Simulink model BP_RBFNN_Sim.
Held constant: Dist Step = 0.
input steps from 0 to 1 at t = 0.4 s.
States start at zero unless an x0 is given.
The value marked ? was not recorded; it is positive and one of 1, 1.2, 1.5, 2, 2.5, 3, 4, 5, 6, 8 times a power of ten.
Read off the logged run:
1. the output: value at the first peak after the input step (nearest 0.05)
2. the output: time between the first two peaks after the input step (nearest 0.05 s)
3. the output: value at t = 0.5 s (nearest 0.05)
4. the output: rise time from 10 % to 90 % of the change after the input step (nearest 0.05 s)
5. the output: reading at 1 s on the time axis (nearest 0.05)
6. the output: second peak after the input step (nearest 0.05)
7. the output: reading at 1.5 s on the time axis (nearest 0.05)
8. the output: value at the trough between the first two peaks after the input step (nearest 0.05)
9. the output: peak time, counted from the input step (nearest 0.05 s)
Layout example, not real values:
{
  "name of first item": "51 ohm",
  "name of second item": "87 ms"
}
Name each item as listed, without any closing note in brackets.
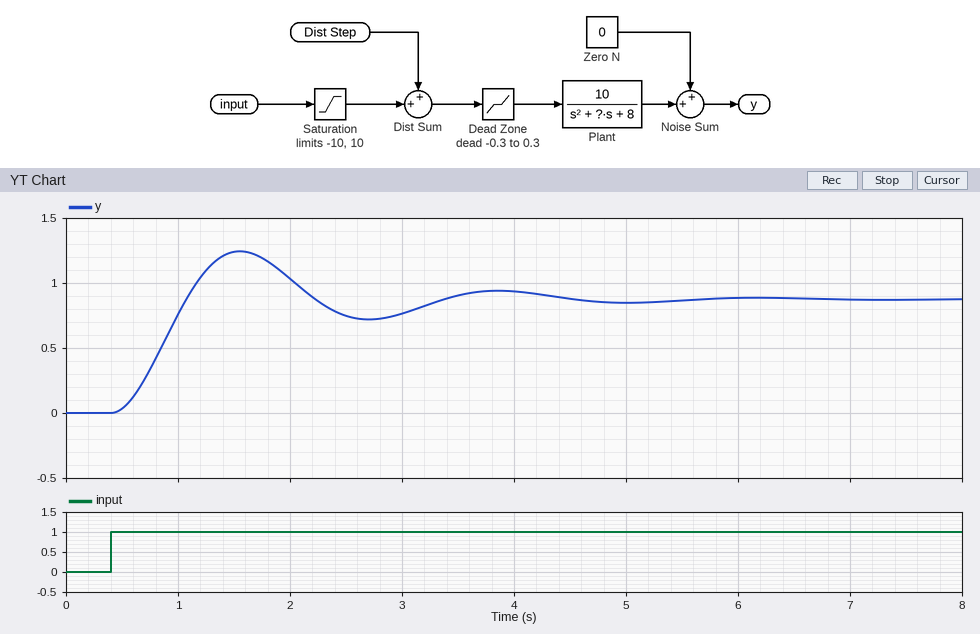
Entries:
{
  "the output: value at the first peak after the input step": "1.25",
  "the output: time between the first two peaks after the input step": "2.30 s",
  "the output: value at t = 0.5 s": "0.05",
  "the output: rise time from 10 % to 90 % of the change after the input step": "0.45 s",
  "the output: reading at 1 s on the time axis": "0.75",
  "the output: second peak after the input step": "0.95",
  "the output: reading at 1.5 s on the time axis": "1.25",
  "the output: value at the trough between the first two peaks after the input step": "0.70",
  "the output: peak time, counted from the input step": "1.15 s"
}
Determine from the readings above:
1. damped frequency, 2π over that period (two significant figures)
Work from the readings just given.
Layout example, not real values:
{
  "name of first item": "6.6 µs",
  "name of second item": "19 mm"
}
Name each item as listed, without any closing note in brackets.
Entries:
{
  "damped frequency, 2π over that period": "2.7 rad/s"
}
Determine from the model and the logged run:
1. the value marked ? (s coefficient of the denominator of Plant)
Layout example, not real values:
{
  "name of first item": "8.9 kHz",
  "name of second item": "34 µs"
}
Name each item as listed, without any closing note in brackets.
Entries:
{
  "the value marked ?": "1.5"
}
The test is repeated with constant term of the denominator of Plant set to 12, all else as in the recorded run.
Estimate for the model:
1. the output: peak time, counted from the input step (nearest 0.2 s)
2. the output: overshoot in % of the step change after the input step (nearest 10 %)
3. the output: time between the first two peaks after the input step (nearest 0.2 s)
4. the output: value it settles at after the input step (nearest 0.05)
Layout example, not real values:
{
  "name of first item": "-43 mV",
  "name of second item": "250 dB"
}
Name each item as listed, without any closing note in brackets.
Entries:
{
  "the output: peak time, counted from the input step": "1.0 s",
  "the output: overshoot in % of the step change after the input step": "50 %",
  "the output: time between the first two peaks after the input step": "1.8 s",
  "the output: value it settles at after the input step": "0.60"
}
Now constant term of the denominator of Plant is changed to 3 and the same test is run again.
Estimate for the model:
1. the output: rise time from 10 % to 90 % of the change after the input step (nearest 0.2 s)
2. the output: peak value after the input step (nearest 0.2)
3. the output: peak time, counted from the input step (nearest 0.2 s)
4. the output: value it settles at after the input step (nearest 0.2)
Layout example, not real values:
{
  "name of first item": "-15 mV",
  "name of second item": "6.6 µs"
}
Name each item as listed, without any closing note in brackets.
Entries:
{
  "the output: rise time from 10 % to 90 % of the change after the input step": "0.8 s",
  "the output: peak value after the input step": "2.8",
  "the output: peak time, counted from the input step": "2.0 s",
  "the output: value it settles at after the input step": "2.4"
}
